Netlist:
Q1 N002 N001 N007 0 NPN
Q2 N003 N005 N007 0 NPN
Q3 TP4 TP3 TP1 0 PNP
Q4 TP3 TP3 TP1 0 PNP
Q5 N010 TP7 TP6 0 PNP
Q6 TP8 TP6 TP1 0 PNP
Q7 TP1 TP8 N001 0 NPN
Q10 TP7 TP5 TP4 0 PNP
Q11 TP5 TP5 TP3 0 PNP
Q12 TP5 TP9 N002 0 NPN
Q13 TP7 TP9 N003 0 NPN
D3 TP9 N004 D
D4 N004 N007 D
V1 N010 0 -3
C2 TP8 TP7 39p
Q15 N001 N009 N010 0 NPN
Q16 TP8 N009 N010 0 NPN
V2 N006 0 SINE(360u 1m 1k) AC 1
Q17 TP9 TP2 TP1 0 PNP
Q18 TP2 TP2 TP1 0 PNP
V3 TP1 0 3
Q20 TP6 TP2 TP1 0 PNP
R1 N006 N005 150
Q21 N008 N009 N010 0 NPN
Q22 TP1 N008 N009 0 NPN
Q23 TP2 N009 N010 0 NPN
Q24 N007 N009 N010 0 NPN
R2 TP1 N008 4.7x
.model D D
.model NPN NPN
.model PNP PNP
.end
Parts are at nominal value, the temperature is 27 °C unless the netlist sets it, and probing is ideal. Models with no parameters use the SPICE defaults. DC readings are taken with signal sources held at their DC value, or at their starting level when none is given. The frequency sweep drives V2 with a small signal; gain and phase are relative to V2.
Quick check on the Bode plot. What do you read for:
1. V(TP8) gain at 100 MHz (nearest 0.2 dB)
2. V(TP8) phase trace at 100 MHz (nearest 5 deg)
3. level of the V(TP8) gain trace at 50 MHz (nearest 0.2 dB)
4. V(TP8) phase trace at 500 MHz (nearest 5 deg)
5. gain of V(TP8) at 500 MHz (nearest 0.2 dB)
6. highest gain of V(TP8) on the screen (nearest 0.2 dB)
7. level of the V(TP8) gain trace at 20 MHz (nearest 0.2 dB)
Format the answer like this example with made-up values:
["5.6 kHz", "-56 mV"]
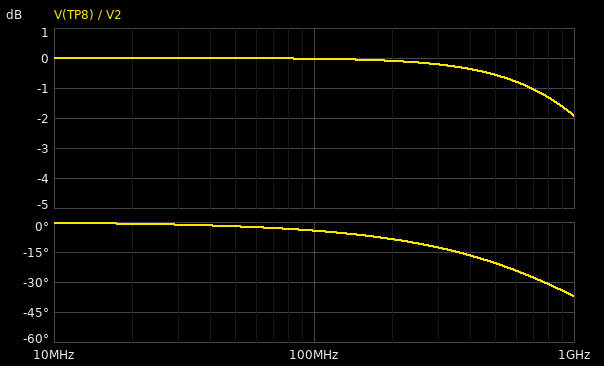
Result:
["0 dB", "-5 deg", "0 dB", "-20 deg", "-0.6 dB", "0 dB", "0 dB"]
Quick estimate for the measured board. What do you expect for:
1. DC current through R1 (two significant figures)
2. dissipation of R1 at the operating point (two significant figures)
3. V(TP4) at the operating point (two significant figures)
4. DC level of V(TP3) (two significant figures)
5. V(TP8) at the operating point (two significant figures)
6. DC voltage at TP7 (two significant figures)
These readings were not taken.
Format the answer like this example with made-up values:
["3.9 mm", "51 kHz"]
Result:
["170 µA", "4.4 µW", "2.2 V", "2.2 V", "910 mV", "1.1 V"]
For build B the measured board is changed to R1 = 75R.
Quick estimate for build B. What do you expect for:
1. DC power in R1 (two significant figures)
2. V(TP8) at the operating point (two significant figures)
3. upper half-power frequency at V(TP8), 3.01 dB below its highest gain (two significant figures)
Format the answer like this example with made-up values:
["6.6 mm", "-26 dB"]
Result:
["2.2 µW", "920 mV", "1.5 GHz"]
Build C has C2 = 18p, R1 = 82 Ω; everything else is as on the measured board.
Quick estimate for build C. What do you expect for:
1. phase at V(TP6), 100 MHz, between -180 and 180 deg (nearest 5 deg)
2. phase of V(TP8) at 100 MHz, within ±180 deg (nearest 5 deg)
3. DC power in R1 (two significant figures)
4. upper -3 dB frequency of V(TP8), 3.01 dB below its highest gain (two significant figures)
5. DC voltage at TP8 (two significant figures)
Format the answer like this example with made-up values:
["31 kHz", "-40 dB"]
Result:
["-90 deg", "0 deg", "2.4 µW", "3.3 GHz", "920 mV"]
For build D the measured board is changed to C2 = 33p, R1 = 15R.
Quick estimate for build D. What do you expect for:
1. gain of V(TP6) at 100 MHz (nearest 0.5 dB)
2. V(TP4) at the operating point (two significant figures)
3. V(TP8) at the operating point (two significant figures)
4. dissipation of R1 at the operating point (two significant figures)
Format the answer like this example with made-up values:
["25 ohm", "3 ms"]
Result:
["-64.5 dB", "2.2 V", "930 mV", "440 nW"]
